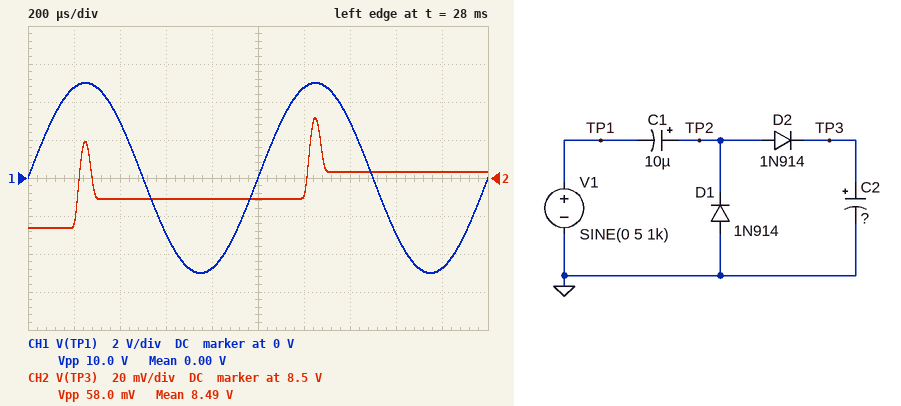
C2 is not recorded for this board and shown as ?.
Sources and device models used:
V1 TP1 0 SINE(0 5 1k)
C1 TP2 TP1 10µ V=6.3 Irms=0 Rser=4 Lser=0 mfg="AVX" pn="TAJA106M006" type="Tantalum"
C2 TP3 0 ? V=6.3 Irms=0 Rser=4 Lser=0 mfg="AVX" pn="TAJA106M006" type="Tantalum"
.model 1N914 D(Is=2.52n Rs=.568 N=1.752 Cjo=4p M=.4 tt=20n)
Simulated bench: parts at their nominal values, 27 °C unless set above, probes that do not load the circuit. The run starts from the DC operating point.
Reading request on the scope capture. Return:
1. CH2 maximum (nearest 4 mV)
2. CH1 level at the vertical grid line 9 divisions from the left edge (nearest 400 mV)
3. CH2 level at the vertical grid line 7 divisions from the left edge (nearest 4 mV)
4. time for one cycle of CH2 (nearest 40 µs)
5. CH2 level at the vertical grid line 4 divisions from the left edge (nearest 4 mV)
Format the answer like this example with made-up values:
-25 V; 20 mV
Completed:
8.532 V; -4.8 V; 8.504 V; 1.00 ms; 8.488 V
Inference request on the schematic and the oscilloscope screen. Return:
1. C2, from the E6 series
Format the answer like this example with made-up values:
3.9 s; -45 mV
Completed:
33 µF
